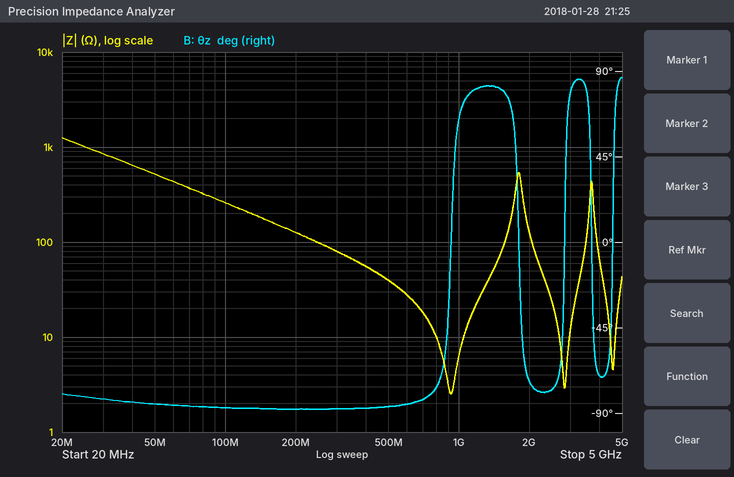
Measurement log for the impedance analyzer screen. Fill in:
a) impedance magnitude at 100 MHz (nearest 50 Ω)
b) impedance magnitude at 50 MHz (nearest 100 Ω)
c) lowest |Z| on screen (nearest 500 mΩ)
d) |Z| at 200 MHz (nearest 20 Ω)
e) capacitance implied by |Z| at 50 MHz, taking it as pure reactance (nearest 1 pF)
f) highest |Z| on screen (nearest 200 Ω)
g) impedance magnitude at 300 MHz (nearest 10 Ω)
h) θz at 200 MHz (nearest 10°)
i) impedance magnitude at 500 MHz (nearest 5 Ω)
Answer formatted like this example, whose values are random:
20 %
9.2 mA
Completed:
250 Ω
500 Ω
2.5 Ω
120 Ω
6 pF
1.2 kΩ
80 Ω
-90°
40 Ω
